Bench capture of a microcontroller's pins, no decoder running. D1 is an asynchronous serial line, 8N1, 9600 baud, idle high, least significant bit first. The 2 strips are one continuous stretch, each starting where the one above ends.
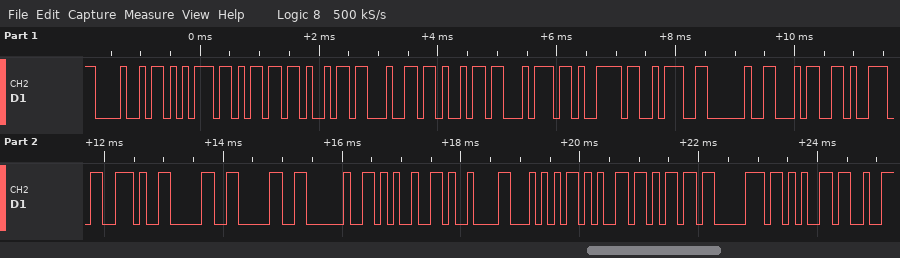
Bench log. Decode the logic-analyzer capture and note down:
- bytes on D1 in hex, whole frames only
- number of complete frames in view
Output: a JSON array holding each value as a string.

["0x48 0x75 0x6D 0x69 0x64 0x69 0x74 0x79 0x3A 0x20 0x34 0x39 0x2E 0x30 0x30 0x20 0x25 0x09 0x54 0x65 0x6D 0x70 0x65", "23"]
